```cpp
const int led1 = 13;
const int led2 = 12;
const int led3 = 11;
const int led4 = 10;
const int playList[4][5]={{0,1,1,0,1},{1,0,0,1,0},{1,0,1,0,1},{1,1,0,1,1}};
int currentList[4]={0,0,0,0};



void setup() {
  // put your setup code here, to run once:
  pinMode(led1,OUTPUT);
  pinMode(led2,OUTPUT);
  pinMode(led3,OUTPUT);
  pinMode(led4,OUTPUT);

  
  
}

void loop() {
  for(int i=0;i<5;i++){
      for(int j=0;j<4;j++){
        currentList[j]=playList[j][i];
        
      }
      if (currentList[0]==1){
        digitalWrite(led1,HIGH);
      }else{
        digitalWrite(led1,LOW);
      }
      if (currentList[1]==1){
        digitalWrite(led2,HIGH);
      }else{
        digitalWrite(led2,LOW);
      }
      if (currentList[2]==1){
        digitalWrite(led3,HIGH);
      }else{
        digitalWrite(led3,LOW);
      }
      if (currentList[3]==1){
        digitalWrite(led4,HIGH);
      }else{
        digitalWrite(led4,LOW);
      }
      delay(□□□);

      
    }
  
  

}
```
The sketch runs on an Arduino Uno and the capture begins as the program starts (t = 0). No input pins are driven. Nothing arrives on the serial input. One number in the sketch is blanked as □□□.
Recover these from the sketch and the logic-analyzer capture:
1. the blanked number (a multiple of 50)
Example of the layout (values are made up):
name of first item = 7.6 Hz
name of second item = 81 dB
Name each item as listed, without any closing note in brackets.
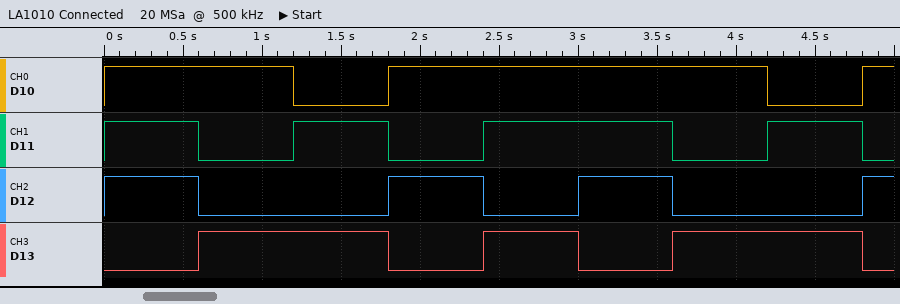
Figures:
the blanked number = 600
